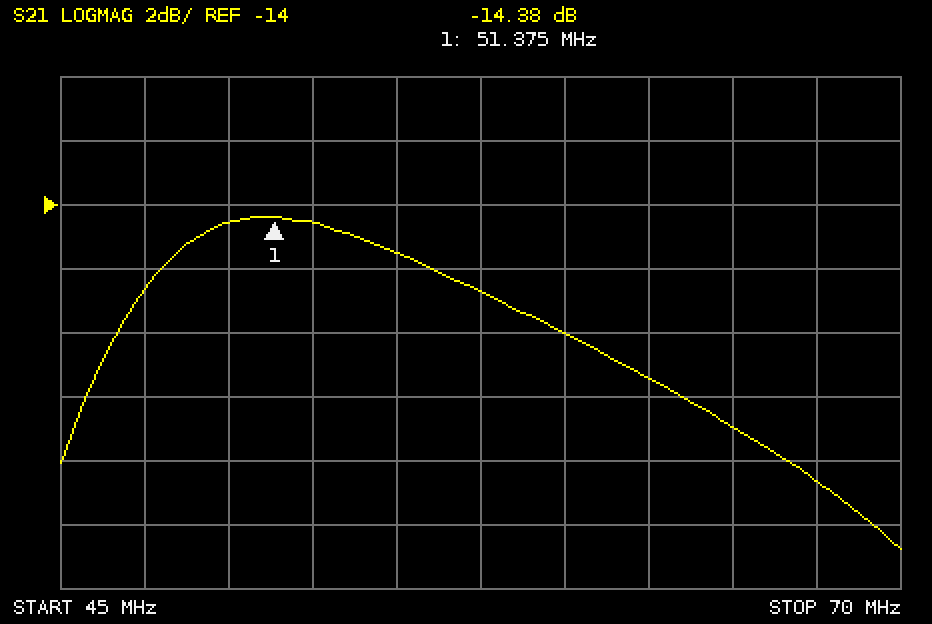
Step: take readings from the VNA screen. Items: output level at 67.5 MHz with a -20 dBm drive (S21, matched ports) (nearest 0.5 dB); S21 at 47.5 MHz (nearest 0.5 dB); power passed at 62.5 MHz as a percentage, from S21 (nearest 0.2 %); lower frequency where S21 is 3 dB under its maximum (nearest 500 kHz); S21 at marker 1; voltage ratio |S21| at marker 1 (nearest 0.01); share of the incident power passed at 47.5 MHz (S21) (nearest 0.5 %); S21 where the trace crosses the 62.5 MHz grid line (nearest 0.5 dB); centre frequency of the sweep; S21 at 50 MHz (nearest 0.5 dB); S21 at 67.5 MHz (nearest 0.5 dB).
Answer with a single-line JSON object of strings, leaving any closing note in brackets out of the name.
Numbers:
{"output level at 67.5 MHz with a -20 dBm drive (S21, matched ports)": "-42.5 dBm", "S21 at 47.5 MHz": "-16.5 dB", "power passed at 62.5 MHz as a percentage, from S21": "1.2 %", "lower frequency where S21 is 3 dB under its maximum": "47.0 MHz", "S21 at marker 1": "-14.38 dB", "voltage ratio |S21| at marker 1": "0.19", "share of the incident power passed at 47.5 MHz (S21)": "2.0 %", "S21 where the trace crosses the 62.5 MHz grid line": "-19.5 dB", "centre frequency of the sweep": "57.5 MHz", "S21 at 50 MHz": "-14.5 dB", "S21 at 67.5 MHz": "-22.5 dB"}
